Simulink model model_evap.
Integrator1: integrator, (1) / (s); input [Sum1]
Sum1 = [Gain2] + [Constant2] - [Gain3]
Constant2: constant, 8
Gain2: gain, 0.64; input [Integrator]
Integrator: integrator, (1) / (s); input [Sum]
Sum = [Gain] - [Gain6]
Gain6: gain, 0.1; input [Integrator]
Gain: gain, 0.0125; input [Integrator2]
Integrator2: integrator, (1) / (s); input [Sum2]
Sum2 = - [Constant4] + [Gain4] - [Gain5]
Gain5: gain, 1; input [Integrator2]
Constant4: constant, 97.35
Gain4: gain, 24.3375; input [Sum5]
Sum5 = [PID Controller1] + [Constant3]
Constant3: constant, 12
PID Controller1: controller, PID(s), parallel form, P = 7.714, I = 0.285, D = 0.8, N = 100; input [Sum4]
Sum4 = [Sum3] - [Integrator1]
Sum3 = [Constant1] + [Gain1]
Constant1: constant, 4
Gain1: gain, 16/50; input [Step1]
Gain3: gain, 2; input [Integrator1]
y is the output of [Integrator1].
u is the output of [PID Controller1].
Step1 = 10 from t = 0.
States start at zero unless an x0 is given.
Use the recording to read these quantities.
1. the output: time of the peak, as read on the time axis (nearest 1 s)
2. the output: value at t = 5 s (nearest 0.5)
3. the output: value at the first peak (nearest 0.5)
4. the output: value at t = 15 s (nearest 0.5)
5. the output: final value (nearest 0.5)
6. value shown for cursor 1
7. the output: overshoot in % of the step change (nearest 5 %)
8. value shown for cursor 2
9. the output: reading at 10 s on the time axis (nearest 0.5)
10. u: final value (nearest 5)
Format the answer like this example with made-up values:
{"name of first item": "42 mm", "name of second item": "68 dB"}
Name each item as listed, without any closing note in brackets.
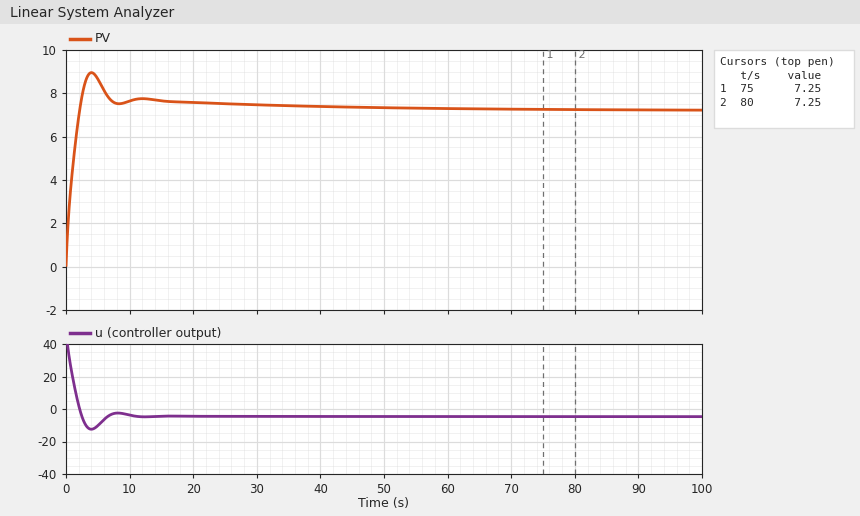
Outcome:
{"the output: time of the peak, as read on the time axis": "4 s", "the output: value at t = 5 s": "8.5", "the output: value at the first peak": "9.0", "the output: value at t = 15 s": "7.5", "the output: final value": "7.0", "value shown for cursor 1": "7.25", "the output: overshoot in % of the step change": "25 %", "value shown for cursor 2": "7.25", "the output: reading at 10 s on the time axis": "7.5", "u: final value": "-5"}
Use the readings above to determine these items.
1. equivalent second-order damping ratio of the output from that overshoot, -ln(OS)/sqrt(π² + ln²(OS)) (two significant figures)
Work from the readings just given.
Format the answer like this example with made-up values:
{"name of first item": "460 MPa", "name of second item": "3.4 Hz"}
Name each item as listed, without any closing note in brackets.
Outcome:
{"equivalent second-order damping ratio of the output from that overshoot, -ln(OS)/sqrt(π² + ln²(OS))": "0.40"}
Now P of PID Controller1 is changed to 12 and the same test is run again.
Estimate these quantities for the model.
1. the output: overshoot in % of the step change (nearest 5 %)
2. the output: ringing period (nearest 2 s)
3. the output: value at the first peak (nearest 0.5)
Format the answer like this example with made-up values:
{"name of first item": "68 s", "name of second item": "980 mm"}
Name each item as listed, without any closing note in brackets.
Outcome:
{"the output: overshoot in % of the step change": "30 %", "the output: ringing period": "6 s", "the output: value at the first peak": "9.5"}
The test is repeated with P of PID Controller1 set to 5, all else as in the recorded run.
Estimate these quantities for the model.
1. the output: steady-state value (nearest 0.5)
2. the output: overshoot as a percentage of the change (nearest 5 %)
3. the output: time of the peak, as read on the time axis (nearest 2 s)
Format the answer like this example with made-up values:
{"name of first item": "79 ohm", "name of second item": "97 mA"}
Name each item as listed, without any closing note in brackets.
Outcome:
{"the output: steady-state value": "7.0", "the output: overshoot as a percentage of the change": "20 %", "the output: time of the peak, as read on the time axis": "6 s"}
